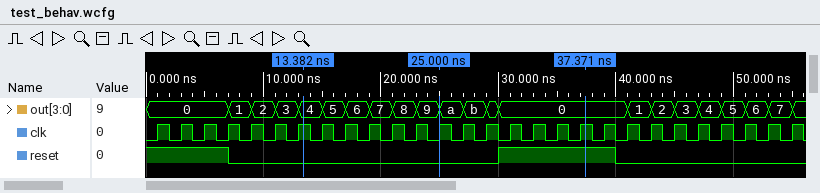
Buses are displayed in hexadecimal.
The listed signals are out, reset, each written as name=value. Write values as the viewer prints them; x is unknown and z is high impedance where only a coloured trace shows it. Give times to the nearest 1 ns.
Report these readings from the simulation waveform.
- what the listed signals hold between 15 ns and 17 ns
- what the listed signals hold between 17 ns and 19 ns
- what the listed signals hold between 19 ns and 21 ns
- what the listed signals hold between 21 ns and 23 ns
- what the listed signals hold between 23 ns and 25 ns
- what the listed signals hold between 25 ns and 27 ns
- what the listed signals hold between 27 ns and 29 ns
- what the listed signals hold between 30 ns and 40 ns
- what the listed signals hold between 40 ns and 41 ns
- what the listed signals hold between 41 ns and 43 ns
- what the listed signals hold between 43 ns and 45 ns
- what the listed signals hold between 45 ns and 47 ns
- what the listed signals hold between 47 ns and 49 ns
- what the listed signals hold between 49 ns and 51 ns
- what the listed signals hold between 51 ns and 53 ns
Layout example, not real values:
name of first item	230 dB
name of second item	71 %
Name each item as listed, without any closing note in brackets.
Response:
what the listed signals hold between 15 ns and 17 ns	out=5, reset=0
what the listed signals hold between 17 ns and 19 ns	out=6, reset=0
what the listed signals hold between 19 ns and 21 ns	out=7, reset=0
what the listed signals hold between 21 ns and 23 ns	out=8, reset=0
what the listed signals hold between 23 ns and 25 ns	out=9, reset=0
what the listed signals hold between 25 ns and 27 ns	out=a, reset=0
what the listed signals hold between 27 ns and 29 ns	out=b, reset=0
what the listed signals hold between 30 ns and 40 ns	out=0, reset=1
what the listed signals hold between 40 ns and 41 ns	out=0, reset=0
what the listed signals hold between 41 ns and 43 ns	out=1, reset=0
what the listed signals hold between 43 ns and 45 ns	out=2, reset=0
what the listed signals hold between 45 ns and 47 ns	out=3, reset=0
what the listed signals hold between 47 ns and 49 ns	out=4, reset=0
what the listed signals hold between 49 ns and 51 ns	out=5, reset=0
what the listed signals hold between 51 ns and 53 ns	out=6, reset=0
